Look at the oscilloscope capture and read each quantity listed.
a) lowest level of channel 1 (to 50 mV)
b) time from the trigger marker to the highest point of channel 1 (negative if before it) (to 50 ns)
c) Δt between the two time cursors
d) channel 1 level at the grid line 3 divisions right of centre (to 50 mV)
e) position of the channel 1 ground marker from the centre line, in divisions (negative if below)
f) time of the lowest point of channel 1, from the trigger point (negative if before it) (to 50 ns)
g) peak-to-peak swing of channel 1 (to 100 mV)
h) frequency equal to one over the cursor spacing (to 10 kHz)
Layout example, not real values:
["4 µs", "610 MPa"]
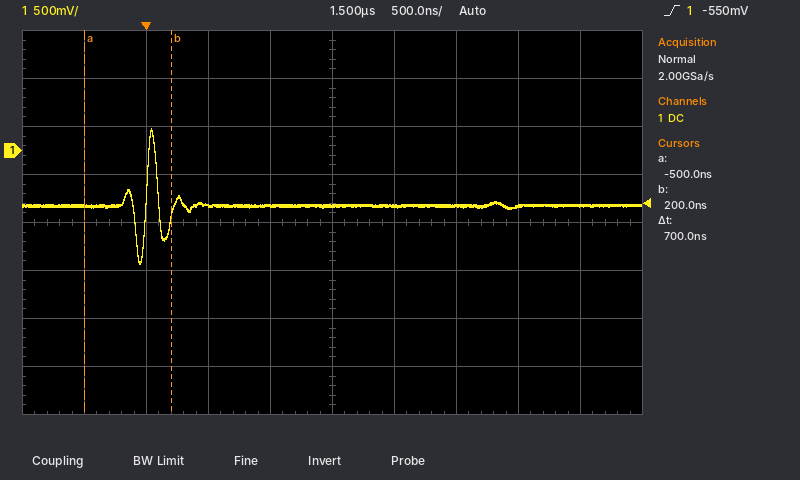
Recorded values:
["-1.20 V", "+50 ns", "700 ns", "-600 mV", "+1.5 div", "-50 ns", "1.40 V", "1.43 MHz"]
